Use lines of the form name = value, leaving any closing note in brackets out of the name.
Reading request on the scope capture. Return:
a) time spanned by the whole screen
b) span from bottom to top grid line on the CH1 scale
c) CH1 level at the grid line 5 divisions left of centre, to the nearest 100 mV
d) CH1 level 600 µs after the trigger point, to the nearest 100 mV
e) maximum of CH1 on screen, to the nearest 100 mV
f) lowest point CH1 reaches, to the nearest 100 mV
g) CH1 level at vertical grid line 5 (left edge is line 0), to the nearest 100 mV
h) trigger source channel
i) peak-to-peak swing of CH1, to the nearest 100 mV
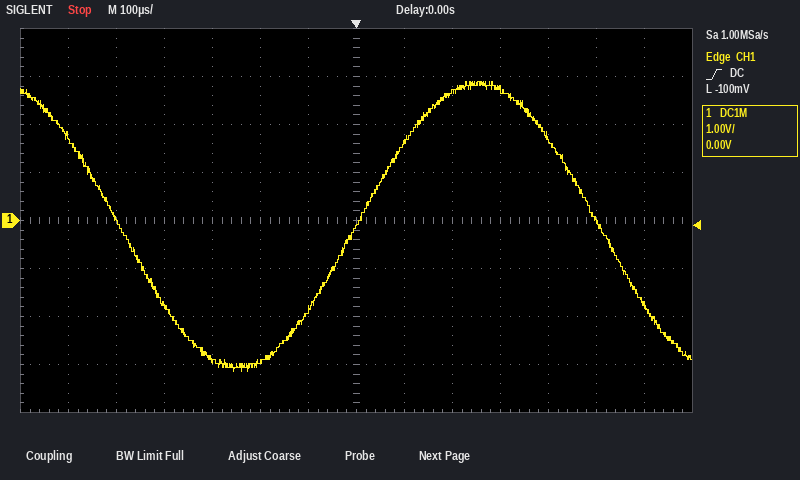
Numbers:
time spanned by the whole screen = 1.4 ms
span from bottom to top grid line on the CH1 scale = 8 V
CH1 level at the grid line 5 divisions left of centre, to the nearest 100 mV = 0.0 V
CH1 level 600 µs after the trigger point, to the nearest 100 mV = -1.8 V
maximum of CH1 on screen, to the nearest 100 mV = 2.9 V
lowest point CH1 reaches, to the nearest 100 mV = -3.1 V
CH1 level at vertical grid line 5 (left edge is line 0), to the nearest 100 mV = -2.9 V
trigger source channel = CH1
peak-to-peak swing of CH1, to the nearest 100 mV = 6.0 V
